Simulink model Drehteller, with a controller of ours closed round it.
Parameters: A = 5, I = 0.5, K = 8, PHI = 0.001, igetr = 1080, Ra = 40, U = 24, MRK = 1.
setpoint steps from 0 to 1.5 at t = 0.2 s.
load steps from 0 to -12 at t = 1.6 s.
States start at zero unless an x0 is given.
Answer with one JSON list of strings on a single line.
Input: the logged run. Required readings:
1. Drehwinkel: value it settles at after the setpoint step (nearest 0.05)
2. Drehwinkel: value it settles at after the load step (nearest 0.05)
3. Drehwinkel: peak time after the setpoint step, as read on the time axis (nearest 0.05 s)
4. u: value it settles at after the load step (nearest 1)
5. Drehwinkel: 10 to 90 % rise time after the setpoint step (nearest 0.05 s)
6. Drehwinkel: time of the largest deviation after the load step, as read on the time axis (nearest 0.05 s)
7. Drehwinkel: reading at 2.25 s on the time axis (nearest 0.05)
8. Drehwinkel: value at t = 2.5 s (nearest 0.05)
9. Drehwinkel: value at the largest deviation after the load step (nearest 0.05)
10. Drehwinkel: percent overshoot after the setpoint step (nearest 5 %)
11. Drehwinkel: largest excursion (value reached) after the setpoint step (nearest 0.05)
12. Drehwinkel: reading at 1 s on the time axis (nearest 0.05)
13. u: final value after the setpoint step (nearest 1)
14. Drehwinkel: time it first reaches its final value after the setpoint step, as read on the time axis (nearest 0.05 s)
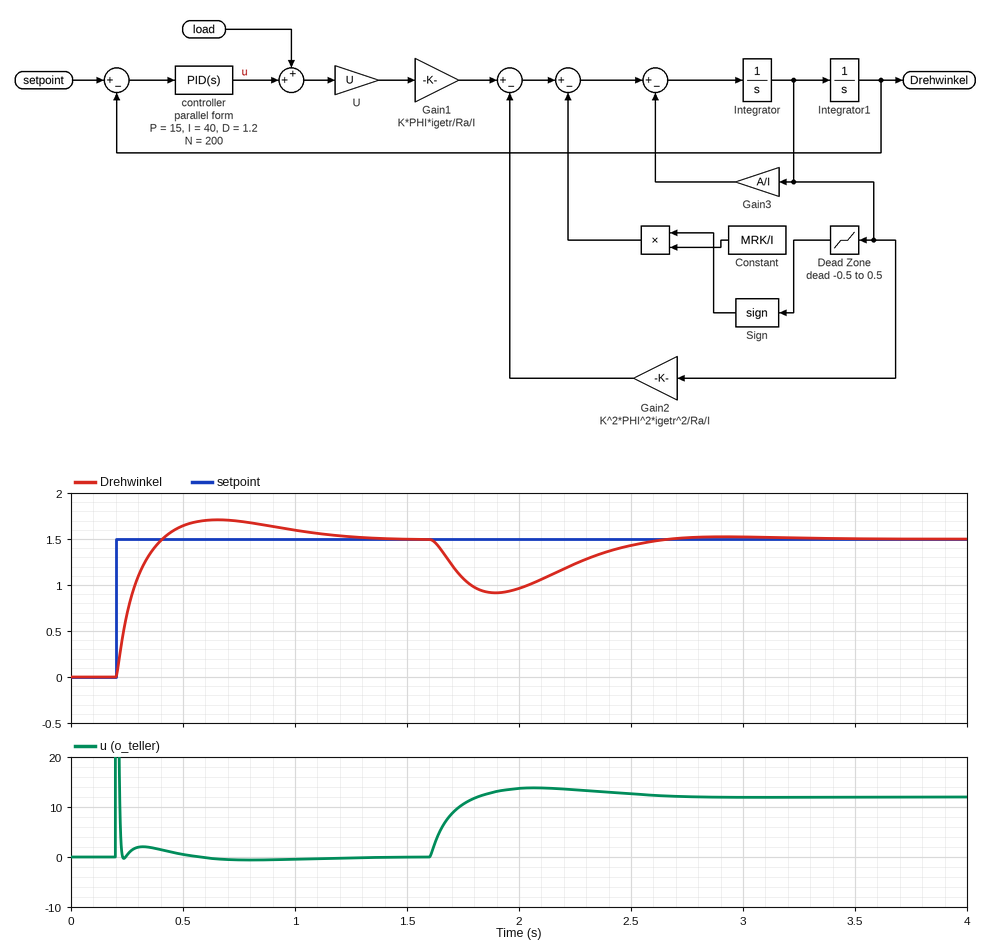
["1.50", "1.50", "0.65 s", "12", "0.15 s", "1.90 s", "1.25", "1.45", "0.90", "15 %", "1.70", "1.60", "0", "0.40 s"]
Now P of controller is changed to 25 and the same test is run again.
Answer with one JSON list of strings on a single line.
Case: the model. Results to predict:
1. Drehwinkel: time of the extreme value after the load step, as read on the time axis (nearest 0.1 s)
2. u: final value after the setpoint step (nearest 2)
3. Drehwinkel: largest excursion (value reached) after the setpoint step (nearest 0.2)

["1.8 s", "0", "1.6"]
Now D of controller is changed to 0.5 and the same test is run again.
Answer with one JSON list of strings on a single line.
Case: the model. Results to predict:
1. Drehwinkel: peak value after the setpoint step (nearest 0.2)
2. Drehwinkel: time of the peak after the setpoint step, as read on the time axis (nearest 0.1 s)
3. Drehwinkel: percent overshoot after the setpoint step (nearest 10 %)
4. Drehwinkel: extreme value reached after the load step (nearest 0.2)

["1.8", "0.5 s", "20 %", "0.8"]
